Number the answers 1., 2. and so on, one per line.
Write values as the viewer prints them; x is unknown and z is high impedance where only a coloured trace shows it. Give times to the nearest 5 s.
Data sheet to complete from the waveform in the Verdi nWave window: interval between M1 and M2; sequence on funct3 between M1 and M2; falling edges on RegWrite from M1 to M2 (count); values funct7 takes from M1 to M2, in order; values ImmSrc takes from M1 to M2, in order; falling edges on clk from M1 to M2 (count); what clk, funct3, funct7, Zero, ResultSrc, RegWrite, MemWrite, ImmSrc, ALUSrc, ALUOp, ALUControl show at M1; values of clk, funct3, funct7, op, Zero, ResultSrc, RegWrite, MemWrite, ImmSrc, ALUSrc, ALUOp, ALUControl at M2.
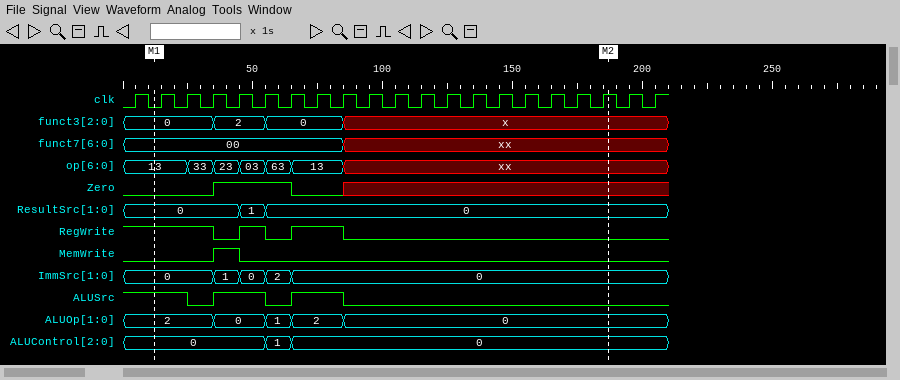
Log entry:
1. 175 s
2. 0, 2, 0, x
3. 3
4. 00, xx
5. 0, 1, 0, 2, 0
6. 17
7. clk=0, funct3=0, funct7=00, Zero=0, ResultSrc=0, RegWrite=1, MemWrite=0, ImmSrc=0, ALUSrc=1, ALUOp=2, ALUControl=0
8. clk=1, funct3=x, funct7=xx, op=xx, Zero=x, ResultSrc=0, RegWrite=0, MemWrite=0, ImmSrc=0, ALUSrc=0, ALUOp=0, ALUControl=0
